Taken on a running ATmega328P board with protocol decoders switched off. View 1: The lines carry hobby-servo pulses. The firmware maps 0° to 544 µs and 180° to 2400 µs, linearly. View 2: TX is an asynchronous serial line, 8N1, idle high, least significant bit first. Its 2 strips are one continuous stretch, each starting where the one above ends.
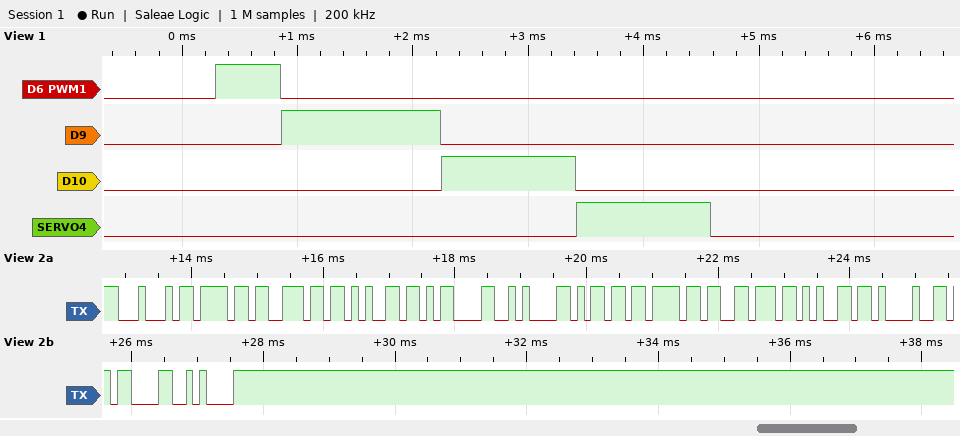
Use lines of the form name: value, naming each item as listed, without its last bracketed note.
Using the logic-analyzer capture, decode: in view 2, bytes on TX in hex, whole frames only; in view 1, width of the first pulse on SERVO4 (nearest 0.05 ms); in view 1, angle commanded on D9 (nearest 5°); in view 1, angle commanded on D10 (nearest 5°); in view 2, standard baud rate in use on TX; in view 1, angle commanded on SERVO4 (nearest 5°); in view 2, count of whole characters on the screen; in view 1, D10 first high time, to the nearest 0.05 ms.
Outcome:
in view 2, bytes on TX in hex, whole frames only: 44 6F 6E 65 0D 0A 6D 6F 76 65 21 0D 0A
in view 1, width of the first pulse on SERVO4: 1.15 ms
in view 1, angle commanded on D9: 80°
in view 1, angle commanded on D10: 60°
in view 2, standard baud rate in use on TX: 9600 baud
in view 1, angle commanded on SERVO4: 60°
in view 2, count of whole characters on the screen: 13
in view 1, D10 first high time, to the nearest 0.05 ms: 1.15 ms
